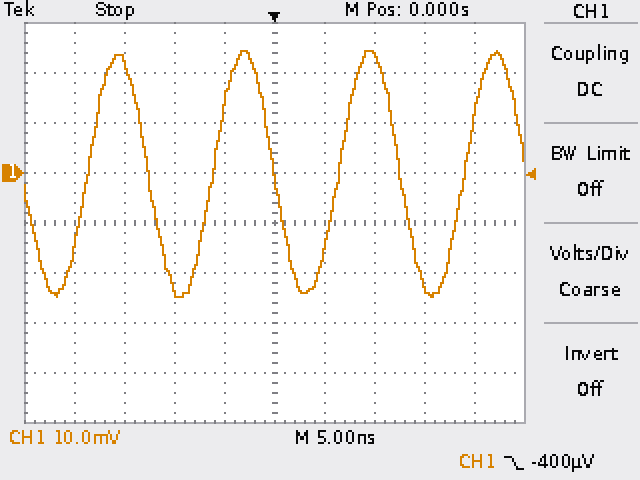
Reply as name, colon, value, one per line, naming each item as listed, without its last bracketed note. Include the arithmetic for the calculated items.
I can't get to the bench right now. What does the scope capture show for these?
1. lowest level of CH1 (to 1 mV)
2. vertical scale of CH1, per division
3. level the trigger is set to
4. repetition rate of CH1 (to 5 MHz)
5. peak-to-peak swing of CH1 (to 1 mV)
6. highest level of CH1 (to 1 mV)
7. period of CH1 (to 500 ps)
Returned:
lowest level of CH1: -25 mV
vertical scale of CH1, per division: 10 mV
level the trigger is set to: -400 µV
repetition rate of CH1: 1 / 12.5 ns ≈ 80 MHz
peak-to-peak swing of CH1: 24 mV − (-25 mV) = 49 mV
highest level of CH1: 24 mV
period of CH1: 12.5 ns
